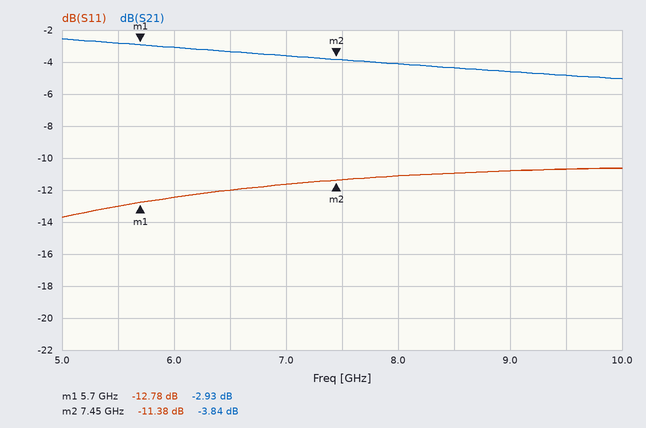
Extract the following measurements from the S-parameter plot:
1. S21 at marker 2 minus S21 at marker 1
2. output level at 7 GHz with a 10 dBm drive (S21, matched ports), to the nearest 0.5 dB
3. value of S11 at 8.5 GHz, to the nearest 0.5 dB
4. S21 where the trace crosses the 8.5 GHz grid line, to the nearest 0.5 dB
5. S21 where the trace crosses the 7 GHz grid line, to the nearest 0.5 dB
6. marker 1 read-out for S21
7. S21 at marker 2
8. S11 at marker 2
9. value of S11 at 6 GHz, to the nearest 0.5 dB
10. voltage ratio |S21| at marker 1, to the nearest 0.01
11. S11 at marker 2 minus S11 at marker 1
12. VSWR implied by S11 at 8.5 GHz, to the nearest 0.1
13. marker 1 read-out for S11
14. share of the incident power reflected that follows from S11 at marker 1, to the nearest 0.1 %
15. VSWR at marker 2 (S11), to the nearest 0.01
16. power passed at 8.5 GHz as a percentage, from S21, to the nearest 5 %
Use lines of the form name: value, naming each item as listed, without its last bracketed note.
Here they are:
S21 at marker 2 minus S21 at marker 1: -0.91 dB
output level at 7 GHz with a 10 dBm drive (S21, matched ports), to the nearest 0.5 dB: 6.5 dBm
value of S11 at 8.5 GHz, to the nearest 0.5 dB: -11.0 dB
S21 where the trace crosses the 8.5 GHz grid line, to the nearest 0.5 dB: -4.5 dB
S21 where the trace crosses the 7 GHz grid line, to the nearest 0.5 dB: -3.5 dB
marker 1 read-out for S21: -2.93 dB
S21 at marker 2: -3.84 dB
S11 at marker 2: -11.38 dB
value of S11 at 6 GHz, to the nearest 0.5 dB: -12.5 dB
voltage ratio |S21| at marker 1, to the nearest 0.01: 0.71
S11 at marker 2 minus S11 at marker 1: 1.40 dB
VSWR implied by S11 at 8.5 GHz, to the nearest 0.1: 1.8
marker 1 read-out for S11: -12.78 dB
share of the incident power reflected that follows from S11 at marker 1, to the nearest 0.1 %: 5.3 %
VSWR at marker 2 (S11), to the nearest 0.01: 1.74
power passed at 8.5 GHz as a percentage, from S21, to the nearest 5 %: 35 %
